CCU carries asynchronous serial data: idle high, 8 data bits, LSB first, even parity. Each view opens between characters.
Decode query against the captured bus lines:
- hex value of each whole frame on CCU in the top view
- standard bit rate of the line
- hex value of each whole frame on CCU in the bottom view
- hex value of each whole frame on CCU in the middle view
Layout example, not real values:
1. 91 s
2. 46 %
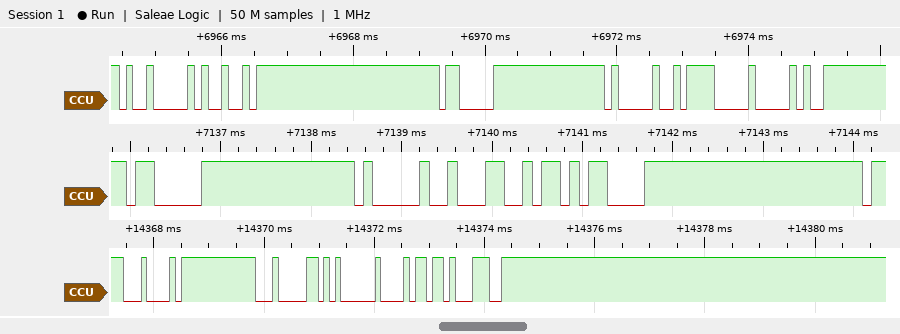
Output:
1. 09, 49, 83, 41, 0F, 50
2. 9600 baud
3. 84, 04, 05, 68, 71
4. 83, 41, 4C, 0D
